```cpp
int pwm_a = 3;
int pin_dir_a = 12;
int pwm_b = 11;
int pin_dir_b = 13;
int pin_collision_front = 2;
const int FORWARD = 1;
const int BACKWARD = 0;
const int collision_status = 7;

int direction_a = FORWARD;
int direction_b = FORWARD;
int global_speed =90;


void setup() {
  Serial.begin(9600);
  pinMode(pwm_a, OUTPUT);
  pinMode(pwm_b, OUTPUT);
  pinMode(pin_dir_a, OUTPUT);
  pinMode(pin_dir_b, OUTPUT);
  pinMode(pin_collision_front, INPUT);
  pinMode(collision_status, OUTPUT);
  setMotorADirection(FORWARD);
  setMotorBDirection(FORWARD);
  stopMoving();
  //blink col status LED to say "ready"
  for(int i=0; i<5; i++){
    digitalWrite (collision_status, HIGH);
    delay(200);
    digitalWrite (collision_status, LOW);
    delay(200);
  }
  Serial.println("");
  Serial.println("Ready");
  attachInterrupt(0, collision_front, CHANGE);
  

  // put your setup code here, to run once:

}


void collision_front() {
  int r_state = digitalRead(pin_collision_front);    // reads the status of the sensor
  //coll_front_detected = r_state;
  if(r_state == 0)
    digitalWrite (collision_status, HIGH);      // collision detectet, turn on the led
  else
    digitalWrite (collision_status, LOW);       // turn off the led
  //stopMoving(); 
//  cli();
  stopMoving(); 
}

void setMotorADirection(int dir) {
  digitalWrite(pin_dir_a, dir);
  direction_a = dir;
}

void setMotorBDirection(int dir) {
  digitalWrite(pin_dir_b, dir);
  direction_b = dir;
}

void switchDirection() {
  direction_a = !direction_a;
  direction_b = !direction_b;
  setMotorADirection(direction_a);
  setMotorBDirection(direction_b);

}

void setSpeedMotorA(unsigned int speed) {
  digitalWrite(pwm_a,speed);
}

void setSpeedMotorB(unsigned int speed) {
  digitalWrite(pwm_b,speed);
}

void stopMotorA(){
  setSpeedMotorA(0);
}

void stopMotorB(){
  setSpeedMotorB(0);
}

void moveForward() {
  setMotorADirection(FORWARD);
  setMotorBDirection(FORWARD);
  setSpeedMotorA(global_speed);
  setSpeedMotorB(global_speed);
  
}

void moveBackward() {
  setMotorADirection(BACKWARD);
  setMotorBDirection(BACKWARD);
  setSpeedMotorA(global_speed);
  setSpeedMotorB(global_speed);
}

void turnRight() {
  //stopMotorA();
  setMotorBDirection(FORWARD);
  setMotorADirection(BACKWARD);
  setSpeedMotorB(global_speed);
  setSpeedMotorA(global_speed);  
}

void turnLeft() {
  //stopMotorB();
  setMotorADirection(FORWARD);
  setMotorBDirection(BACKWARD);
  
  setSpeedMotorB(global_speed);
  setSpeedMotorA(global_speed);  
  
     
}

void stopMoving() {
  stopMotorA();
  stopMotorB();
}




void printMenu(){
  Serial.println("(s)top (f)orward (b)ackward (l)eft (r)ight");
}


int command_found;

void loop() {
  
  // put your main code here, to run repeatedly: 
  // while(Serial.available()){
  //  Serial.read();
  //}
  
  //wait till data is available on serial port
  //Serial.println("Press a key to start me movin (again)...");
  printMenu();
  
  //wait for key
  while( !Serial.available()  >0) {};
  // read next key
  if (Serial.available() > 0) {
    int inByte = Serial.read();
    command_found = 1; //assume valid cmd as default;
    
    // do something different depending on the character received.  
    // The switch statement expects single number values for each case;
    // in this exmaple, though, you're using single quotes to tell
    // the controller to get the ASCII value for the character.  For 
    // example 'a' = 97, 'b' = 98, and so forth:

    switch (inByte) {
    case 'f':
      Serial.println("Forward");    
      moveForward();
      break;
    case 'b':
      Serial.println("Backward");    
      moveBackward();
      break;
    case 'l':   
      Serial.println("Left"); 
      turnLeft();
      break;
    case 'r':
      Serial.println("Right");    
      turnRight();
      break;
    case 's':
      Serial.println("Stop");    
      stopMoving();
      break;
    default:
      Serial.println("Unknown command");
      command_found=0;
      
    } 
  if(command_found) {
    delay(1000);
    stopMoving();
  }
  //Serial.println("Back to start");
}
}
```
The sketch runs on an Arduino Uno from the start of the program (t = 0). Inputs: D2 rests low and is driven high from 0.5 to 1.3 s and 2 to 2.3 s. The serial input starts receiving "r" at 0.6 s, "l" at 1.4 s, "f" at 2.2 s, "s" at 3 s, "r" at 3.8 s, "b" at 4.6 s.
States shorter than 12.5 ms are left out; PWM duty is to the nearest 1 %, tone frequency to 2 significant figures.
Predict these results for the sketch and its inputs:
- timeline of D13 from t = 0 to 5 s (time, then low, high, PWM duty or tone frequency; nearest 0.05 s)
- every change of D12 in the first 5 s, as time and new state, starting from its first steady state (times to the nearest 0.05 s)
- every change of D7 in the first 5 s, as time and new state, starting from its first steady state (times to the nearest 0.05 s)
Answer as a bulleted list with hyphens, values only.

- 0 s high; 3 s low; 4 s high
- 0 s high; 2 s low; 3 s high
- 0 s high; 0.2 s low; 0.4 s high; 0.6 s low; 0.8 s high; 1 s low; 1.2 s high; 1.4 s low; 1.6 s high; 1.8 s low; 2.3 s high
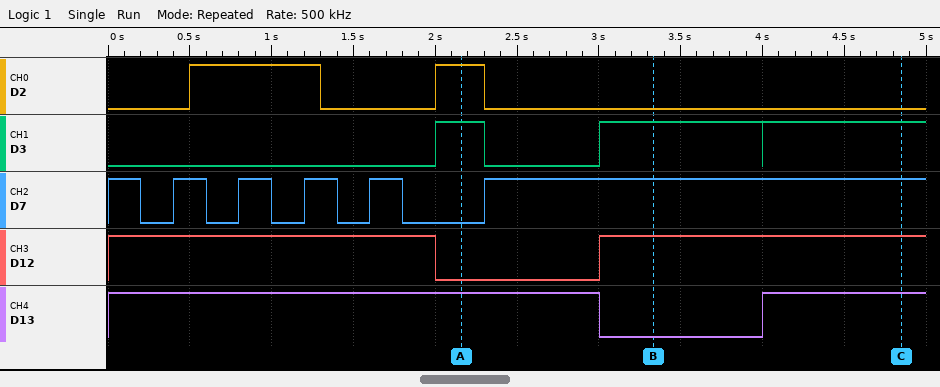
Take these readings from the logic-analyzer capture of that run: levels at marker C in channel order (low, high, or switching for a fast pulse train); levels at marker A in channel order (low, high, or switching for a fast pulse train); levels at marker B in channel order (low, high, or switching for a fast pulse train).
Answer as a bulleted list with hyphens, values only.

- D2 low, D3 high, D7 high, D12 high, D13 high
- D2 high, D3 high, D7 low, D12 low, D13 high
- D2 low, D3 high, D7 high, D12 high, D13 low
